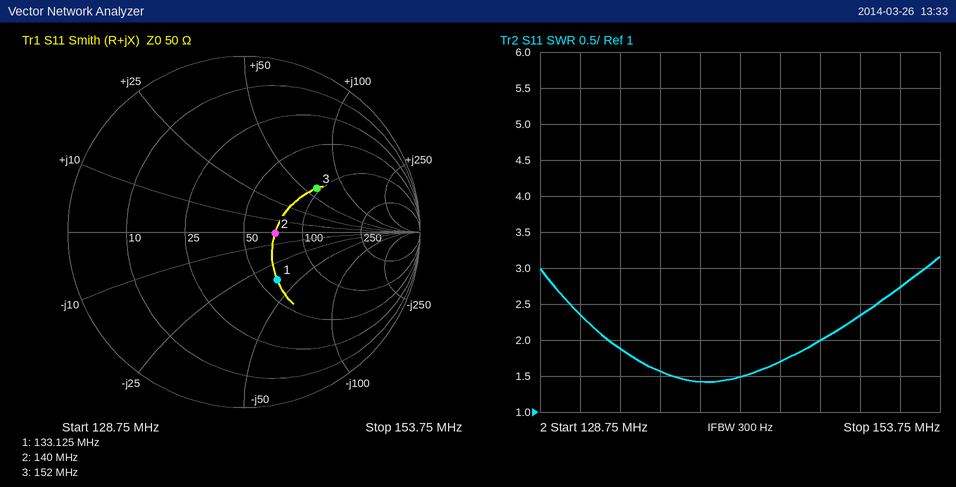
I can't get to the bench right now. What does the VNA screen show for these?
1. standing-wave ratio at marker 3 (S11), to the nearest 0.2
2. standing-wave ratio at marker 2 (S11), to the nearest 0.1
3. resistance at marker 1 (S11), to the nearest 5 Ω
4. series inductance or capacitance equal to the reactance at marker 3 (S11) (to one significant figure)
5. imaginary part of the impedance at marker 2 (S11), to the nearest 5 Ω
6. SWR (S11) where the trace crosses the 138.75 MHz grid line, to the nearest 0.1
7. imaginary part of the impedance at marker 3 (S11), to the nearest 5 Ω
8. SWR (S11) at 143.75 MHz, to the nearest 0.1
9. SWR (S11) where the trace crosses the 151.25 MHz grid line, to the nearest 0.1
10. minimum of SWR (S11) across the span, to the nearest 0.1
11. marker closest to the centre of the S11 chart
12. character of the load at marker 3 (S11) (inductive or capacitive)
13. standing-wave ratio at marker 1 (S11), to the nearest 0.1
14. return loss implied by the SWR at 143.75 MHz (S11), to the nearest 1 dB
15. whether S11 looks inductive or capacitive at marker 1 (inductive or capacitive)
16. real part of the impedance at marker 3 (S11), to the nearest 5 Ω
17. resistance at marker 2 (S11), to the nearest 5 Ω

2.8
1.4
60 Ω
60 nH
0 Ω
1.4
+60 Ω
1.7
2.7
1.4
marker 2
inductive
2.0
12 dB
capacitive
95 Ω
70 Ω
